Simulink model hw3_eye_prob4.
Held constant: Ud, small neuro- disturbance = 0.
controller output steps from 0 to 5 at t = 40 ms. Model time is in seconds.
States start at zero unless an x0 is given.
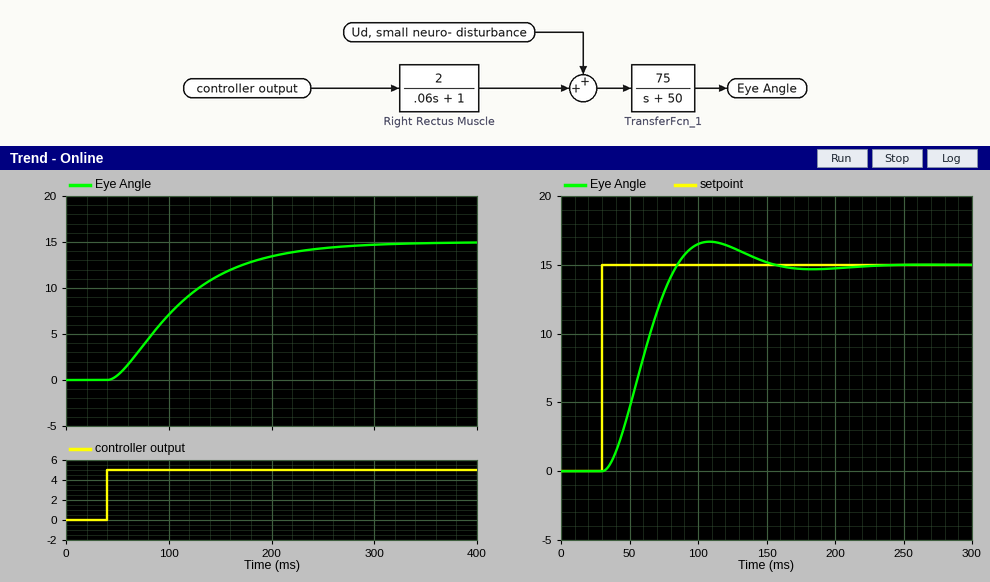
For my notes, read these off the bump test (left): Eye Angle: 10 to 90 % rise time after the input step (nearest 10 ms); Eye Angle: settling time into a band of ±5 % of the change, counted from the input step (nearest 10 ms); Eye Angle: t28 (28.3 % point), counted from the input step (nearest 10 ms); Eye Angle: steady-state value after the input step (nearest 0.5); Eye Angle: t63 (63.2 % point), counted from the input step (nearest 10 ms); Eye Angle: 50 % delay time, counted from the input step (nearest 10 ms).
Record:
140 ms
200 ms
40 ms
15.0
80 ms
60 ms
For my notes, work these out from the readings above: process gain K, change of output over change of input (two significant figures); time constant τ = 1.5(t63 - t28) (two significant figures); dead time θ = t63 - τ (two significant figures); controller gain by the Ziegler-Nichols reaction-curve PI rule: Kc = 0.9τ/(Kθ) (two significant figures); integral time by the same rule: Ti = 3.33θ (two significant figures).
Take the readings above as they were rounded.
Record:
3.0
60 ms
20 ms
0.90
67 ms
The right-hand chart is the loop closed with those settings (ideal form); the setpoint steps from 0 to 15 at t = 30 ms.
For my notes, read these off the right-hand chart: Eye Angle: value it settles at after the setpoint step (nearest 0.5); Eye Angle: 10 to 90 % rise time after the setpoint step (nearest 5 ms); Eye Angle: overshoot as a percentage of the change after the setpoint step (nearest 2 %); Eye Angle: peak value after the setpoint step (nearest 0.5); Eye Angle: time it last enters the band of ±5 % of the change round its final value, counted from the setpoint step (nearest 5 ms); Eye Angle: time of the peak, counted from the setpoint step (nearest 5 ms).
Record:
15.0
35 ms
12 %
16.5
105 ms
80 ms
